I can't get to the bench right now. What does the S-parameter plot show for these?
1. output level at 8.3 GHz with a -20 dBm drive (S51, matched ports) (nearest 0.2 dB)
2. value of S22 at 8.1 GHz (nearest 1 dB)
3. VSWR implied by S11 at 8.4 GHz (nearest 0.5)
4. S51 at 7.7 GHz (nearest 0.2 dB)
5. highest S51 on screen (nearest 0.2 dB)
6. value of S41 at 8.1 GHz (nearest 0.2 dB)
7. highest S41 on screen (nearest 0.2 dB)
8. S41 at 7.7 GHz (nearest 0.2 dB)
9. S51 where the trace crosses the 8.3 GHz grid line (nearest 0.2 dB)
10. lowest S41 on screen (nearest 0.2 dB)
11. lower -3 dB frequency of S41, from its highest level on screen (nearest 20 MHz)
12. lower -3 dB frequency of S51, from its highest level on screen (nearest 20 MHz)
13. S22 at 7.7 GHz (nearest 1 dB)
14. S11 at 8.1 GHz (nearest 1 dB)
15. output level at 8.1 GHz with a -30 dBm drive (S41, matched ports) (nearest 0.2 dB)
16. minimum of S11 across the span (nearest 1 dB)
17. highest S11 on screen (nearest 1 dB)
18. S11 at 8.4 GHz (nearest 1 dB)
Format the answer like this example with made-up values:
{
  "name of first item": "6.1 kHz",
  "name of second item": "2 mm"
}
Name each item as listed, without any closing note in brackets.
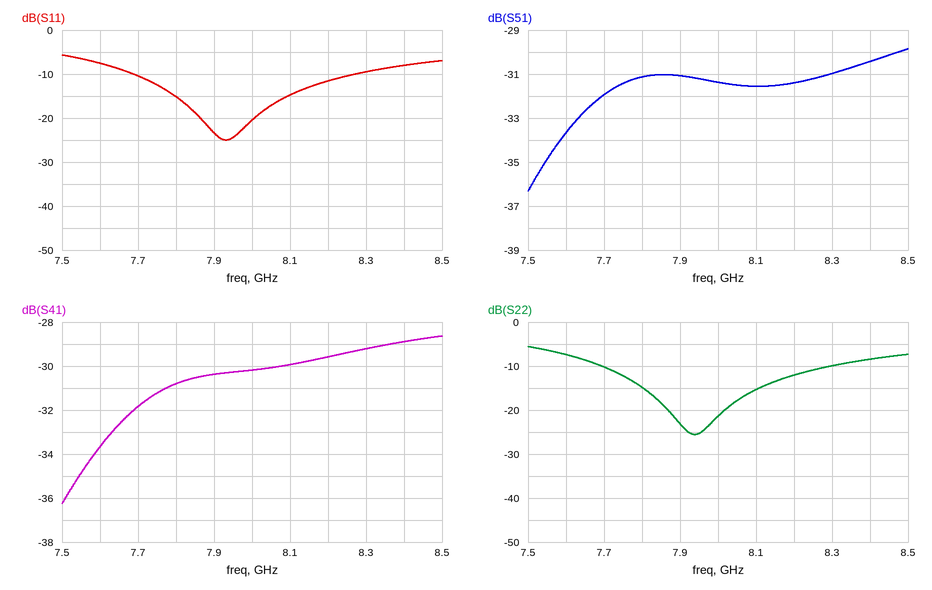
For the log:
{
  "output level at 8.3 GHz with a -20 dBm drive (S51, matched ports)": "-51.0 dBm",
  "value of S22 at 8.1 GHz": "-15 dB",
  "VSWR implied by S11 at 8.4 GHz": "2.5",
  "S51 at 7.7 GHz": "-32.0 dB",
  "highest S51 on screen": "-29.8 dB",
  "value of S41 at 8.1 GHz": "-30.0 dB",
  "highest S41 on screen": "-28.6 dB",
  "S41 at 7.7 GHz": "-31.8 dB",
  "S51 where the trace crosses the 8.3 GHz grid line": "-31.0 dB",
  "lowest S41 on screen": "-36.2 dB",
  "lower -3 dB frequency of S41, from its highest level on screen": "7.72 GHz",
  "lower -3 dB frequency of S51, from its highest level on screen": "7.64 GHz",
  "S22 at 7.7 GHz": "-10 dB",
  "S11 at 8.1 GHz": "-15 dB",
  "output level at 8.1 GHz with a -30 dBm drive (S41, matched ports)": "-60.0 dBm",
  "minimum of S11 across the span": "-25 dB",
  "highest S11 on screen": "-6 dB",
  "S11 at 8.4 GHz": "-8 dB"
}
